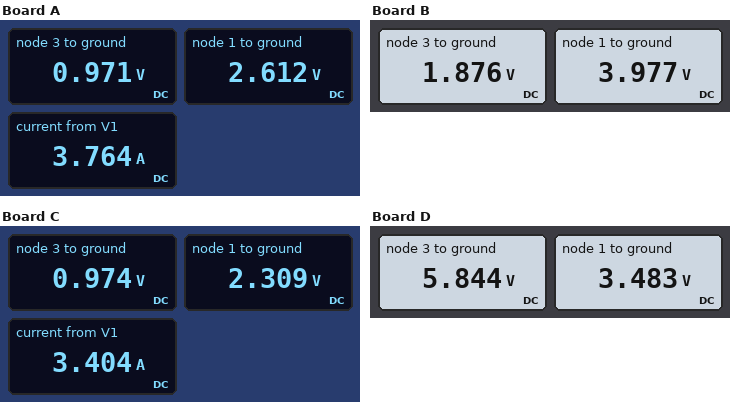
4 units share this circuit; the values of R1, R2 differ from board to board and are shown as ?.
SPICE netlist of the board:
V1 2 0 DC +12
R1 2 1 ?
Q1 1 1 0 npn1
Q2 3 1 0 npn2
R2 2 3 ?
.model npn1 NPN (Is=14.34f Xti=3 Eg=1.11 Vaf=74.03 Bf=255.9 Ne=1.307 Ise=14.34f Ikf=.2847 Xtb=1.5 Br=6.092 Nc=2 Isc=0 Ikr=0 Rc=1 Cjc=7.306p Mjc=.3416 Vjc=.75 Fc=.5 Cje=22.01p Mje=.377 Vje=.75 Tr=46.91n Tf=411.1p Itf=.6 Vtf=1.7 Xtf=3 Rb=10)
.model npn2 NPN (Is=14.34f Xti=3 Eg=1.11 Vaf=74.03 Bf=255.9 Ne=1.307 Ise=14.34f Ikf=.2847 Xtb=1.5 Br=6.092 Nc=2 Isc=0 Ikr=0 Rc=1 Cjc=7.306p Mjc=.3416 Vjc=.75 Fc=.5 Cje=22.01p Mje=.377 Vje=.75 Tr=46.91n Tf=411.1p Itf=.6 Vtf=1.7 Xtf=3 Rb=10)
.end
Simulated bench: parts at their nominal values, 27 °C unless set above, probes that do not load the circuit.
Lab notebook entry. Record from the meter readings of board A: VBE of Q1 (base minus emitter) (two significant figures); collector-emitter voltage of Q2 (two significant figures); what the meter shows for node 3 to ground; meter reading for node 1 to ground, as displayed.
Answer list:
2.6 V
970 mV
0.971 V
2.612 V
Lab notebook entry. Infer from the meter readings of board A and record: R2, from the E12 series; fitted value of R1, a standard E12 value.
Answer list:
12 Ω
3.3 Ω
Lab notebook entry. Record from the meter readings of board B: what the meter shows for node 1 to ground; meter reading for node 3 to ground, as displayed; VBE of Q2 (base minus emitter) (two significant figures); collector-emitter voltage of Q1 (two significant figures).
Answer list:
3.977 V
1.876 V
4.0 V
4.0 V
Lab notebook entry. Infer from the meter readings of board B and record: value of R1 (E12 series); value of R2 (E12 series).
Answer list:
1.8 Ω
5.6 Ω
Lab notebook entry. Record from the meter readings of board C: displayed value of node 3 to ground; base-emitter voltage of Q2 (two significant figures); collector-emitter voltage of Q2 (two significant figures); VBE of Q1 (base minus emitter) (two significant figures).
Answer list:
0.974 V
2.3 V
970 mV
2.3 V
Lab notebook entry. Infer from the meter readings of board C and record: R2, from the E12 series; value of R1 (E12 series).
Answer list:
12 Ω
3.9 Ω
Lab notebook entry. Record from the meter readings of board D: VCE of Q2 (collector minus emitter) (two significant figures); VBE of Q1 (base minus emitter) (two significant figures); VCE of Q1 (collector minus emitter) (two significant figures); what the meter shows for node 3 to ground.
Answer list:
5.8 V
3.5 V
3.5 V
5.844 V
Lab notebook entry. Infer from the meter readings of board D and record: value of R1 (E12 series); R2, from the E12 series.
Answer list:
2.2 Ω
1.5 Ω
